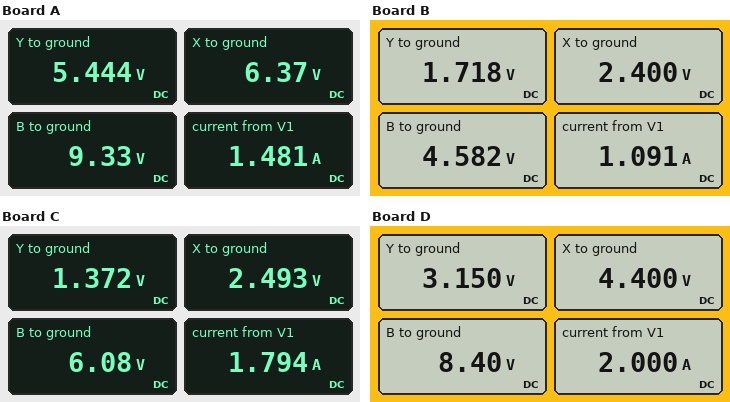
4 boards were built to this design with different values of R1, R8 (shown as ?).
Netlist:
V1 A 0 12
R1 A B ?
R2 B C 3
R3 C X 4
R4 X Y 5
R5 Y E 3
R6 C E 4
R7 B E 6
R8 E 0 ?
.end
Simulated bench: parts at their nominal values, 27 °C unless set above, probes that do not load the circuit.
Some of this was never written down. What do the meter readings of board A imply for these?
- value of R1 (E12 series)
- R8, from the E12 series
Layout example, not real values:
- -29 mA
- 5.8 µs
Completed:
- 1.8 Ω
- 3.3 Ω
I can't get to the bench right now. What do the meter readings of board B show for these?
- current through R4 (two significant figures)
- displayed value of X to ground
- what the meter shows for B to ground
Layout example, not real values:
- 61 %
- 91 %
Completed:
- 140 mA
- 2.400 V
- 4.582 V
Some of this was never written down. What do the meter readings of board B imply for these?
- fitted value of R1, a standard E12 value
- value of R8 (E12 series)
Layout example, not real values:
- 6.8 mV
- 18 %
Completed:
- 6.8 Ω
- 1.2 Ω
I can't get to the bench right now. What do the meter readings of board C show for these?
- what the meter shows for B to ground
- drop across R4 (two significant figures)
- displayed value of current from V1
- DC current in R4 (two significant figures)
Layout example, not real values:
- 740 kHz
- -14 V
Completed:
- 6.08 V
- 1.1 V
- 1.794 A
- 220 mA
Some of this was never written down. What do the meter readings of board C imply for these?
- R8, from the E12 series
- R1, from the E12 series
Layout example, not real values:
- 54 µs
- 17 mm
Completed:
- 0.39 Ω
- 3.3 Ω
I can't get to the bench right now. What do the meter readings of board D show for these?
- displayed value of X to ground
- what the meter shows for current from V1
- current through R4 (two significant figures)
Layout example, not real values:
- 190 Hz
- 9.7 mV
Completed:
- 4.400 V
- 2.000 A
- 250 mA
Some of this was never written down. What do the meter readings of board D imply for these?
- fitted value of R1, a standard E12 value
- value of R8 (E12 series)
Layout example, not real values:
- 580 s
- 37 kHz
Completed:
- 1.8 Ω
- 1.2 Ω
